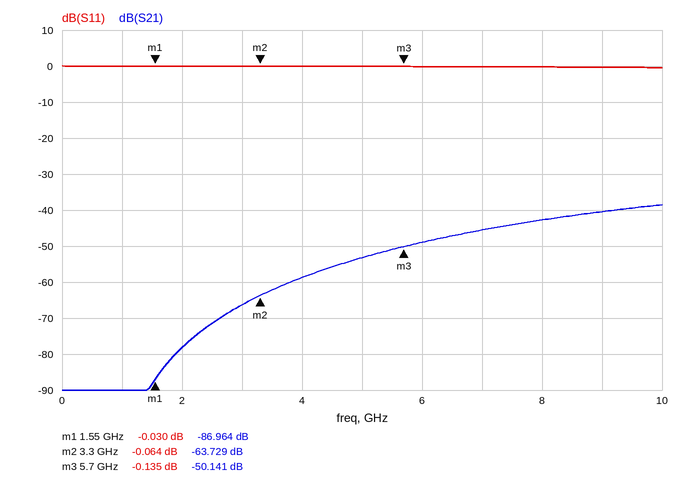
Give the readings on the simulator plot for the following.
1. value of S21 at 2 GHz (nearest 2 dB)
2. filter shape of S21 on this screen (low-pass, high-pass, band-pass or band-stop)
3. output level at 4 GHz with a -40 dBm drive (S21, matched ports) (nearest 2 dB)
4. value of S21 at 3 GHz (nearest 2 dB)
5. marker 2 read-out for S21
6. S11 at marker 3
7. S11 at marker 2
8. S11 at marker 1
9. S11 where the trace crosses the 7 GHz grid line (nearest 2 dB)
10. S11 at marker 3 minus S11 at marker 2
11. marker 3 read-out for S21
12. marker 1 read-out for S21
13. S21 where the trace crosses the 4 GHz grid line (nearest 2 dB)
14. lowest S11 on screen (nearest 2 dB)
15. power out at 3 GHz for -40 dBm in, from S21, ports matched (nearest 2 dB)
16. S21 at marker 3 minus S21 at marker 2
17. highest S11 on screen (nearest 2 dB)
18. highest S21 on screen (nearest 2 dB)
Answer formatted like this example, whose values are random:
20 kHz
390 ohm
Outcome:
-78 dB
high-pass
-98 dBm
-66 dB
-63.729 dB
-0.135 dB
-0.064 dB
-0.030 dB
0 dB
-0.071 dB
-50.141 dB
-86.964 dB
-58 dB
0 dB
-106 dBm
13.588 dB
0 dB
-38 dB
